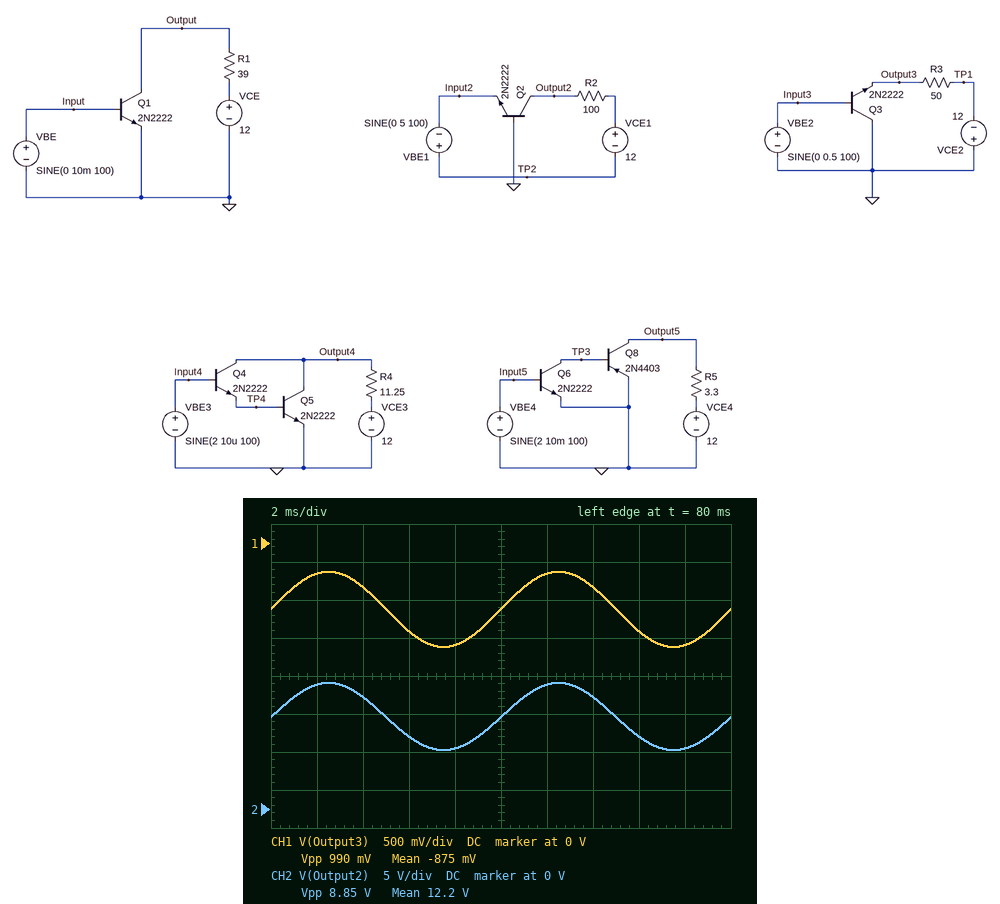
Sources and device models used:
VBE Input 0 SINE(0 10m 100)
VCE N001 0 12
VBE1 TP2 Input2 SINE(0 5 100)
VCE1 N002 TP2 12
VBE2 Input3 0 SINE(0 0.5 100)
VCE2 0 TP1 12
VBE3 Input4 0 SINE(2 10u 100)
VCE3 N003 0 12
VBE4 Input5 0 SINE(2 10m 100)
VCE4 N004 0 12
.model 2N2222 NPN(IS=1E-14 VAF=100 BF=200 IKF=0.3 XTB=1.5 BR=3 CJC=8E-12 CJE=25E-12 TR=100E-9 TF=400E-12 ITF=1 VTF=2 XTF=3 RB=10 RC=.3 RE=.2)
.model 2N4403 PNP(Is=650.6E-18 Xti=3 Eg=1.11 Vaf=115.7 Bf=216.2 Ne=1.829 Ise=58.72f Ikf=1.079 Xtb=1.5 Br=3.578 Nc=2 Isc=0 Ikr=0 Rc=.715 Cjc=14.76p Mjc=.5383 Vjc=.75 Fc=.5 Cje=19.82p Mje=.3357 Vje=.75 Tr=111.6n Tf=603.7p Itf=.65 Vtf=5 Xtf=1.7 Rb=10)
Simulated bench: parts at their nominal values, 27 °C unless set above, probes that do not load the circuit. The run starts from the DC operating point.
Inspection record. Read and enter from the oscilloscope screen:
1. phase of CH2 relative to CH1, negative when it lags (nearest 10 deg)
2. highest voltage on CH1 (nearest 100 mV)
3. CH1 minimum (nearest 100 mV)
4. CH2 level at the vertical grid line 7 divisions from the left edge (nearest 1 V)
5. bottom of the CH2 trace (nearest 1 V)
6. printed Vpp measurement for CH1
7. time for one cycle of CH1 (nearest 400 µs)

0 deg
-400 mV
-1.4 V
15 V
8 V
990 mV
10.0 ms
